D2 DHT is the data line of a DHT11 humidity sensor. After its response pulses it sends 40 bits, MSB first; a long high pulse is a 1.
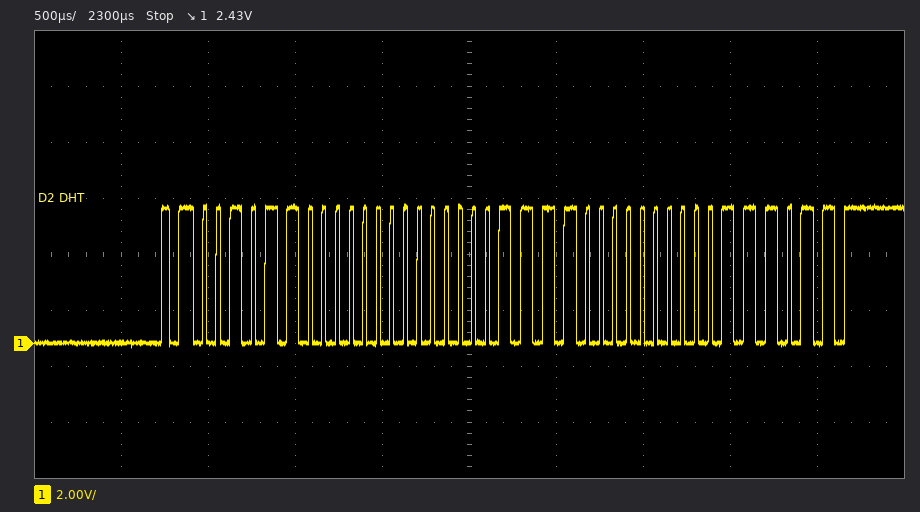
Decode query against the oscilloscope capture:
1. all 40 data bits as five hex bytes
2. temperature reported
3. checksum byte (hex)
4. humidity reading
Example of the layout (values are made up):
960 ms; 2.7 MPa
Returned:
2C 00 0F 00 3B; 15.0 °C; 0x3B; 44 %
